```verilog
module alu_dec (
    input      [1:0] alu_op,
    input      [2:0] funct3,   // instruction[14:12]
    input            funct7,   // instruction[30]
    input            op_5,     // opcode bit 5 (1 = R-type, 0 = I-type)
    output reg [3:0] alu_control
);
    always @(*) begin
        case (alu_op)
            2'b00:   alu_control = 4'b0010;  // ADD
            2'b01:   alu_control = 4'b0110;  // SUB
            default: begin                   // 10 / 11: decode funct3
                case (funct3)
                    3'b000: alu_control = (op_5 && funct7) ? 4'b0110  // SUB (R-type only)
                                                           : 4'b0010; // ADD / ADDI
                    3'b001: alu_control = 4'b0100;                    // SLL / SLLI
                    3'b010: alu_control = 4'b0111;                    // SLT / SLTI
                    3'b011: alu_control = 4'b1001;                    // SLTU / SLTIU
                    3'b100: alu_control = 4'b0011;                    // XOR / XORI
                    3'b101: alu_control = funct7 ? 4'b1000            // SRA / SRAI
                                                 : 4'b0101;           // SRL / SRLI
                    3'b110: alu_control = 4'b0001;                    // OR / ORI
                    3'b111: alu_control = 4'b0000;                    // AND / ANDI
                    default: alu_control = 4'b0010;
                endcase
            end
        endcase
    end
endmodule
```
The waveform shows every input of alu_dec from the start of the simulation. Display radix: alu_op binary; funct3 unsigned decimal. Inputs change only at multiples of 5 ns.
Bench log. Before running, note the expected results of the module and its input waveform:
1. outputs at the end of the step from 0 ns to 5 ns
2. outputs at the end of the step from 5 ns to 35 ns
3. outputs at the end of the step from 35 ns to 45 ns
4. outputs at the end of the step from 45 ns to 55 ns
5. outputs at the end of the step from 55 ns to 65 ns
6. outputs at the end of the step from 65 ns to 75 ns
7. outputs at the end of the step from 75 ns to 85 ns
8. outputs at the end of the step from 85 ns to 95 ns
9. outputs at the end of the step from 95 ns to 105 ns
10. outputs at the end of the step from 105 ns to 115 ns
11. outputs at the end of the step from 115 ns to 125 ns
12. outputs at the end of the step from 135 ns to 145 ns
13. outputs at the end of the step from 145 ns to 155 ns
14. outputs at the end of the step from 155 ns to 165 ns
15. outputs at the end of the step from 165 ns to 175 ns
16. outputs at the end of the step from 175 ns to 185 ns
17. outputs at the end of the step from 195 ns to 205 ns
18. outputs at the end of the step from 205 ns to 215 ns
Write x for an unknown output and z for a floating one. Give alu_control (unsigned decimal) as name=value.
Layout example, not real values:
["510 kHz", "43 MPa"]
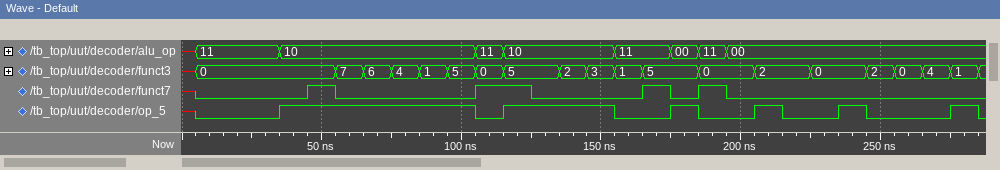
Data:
["alu_control=x", "alu_control=2", "alu_control=2", "alu_control=6", "alu_control=0", "alu_control=1", "alu_control=3", "alu_control=4", "alu_control=5", "alu_control=2", "alu_control=8", "alu_control=7", "alu_control=9", "alu_control=4", "alu_control=8", "alu_control=2", "alu_control=2", "alu_control=2"]
